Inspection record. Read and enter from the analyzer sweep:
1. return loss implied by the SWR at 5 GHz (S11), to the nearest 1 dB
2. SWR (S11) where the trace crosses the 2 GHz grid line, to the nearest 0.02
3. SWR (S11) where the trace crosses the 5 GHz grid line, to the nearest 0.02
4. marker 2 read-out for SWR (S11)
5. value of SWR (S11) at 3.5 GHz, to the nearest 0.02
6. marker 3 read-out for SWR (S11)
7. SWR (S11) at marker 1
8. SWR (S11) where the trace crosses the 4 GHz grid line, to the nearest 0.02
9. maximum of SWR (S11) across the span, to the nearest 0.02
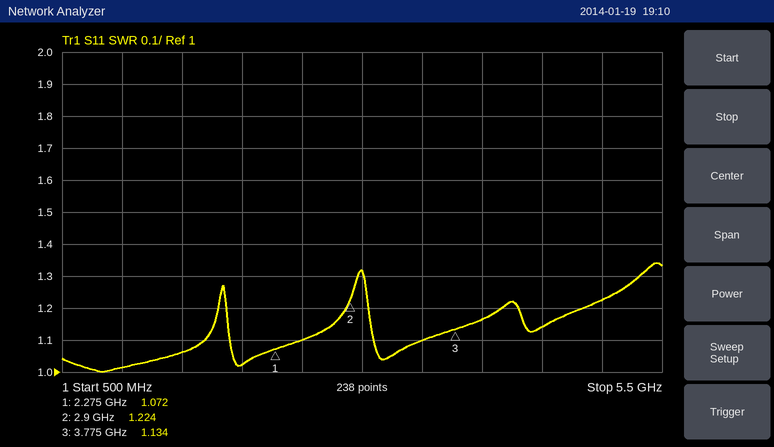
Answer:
20 dB
1.02
1.22
1.224
1.10
1.134
1.072
1.16
1.34
